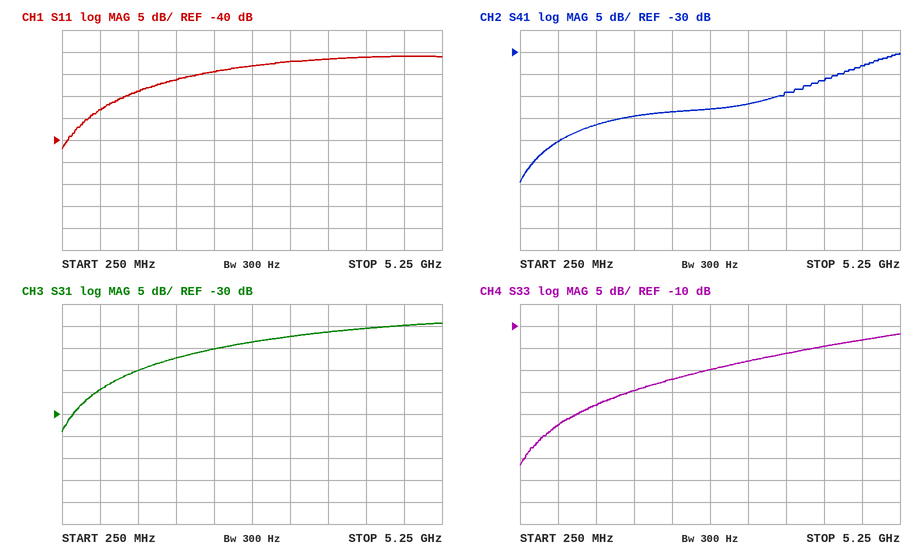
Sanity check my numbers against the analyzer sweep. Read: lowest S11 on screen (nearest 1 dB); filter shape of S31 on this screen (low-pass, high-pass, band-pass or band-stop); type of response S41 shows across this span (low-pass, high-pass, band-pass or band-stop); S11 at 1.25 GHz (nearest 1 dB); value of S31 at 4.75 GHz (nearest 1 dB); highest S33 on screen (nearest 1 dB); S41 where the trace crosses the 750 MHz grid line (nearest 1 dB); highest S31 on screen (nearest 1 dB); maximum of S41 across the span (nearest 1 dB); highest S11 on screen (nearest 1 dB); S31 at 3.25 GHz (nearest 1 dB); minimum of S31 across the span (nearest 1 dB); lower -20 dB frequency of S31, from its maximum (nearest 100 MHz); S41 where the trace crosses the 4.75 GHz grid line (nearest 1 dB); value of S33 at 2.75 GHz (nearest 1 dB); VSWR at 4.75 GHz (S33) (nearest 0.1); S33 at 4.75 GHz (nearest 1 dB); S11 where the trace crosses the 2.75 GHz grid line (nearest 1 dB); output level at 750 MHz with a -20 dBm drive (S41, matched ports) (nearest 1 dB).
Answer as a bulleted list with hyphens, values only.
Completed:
- -42 dB
- high-pass
- high-pass
- -29 dB
- -10 dB
- -12 dB
- -50 dB
- -9 dB
- -30 dB
- -21 dB
- -12 dB
- -34 dB
- 400 MHz
- -33 dB
- -20 dB
- 1.6
- -13 dB
- -23 dB
- -70 dBm
